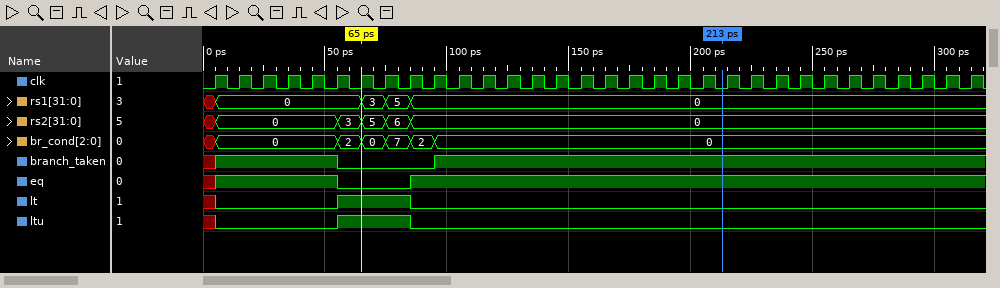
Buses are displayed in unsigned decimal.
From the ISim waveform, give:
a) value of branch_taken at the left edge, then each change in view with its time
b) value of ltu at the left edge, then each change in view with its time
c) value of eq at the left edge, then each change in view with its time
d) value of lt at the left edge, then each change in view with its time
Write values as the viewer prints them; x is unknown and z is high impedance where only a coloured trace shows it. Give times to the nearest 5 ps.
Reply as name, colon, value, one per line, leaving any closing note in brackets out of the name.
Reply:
value of branch_taken at the left edge, then each change in view with its time: x, 1 at 5 ps, 0 at 55 ps, 1 at 95 ps
value of ltu at the left edge, then each change in view with its time: x, 0 at 5 ps, 1 at 55 ps, 0 at 85 ps
value of eq at the left edge, then each change in view with its time: x, 1 at 5 ps, 0 at 55 ps, 1 at 85 ps
value of lt at the left edge, then each change in view with its time: x, 0 at 5 ps, 1 at 55 ps, 0 at 85 ps
